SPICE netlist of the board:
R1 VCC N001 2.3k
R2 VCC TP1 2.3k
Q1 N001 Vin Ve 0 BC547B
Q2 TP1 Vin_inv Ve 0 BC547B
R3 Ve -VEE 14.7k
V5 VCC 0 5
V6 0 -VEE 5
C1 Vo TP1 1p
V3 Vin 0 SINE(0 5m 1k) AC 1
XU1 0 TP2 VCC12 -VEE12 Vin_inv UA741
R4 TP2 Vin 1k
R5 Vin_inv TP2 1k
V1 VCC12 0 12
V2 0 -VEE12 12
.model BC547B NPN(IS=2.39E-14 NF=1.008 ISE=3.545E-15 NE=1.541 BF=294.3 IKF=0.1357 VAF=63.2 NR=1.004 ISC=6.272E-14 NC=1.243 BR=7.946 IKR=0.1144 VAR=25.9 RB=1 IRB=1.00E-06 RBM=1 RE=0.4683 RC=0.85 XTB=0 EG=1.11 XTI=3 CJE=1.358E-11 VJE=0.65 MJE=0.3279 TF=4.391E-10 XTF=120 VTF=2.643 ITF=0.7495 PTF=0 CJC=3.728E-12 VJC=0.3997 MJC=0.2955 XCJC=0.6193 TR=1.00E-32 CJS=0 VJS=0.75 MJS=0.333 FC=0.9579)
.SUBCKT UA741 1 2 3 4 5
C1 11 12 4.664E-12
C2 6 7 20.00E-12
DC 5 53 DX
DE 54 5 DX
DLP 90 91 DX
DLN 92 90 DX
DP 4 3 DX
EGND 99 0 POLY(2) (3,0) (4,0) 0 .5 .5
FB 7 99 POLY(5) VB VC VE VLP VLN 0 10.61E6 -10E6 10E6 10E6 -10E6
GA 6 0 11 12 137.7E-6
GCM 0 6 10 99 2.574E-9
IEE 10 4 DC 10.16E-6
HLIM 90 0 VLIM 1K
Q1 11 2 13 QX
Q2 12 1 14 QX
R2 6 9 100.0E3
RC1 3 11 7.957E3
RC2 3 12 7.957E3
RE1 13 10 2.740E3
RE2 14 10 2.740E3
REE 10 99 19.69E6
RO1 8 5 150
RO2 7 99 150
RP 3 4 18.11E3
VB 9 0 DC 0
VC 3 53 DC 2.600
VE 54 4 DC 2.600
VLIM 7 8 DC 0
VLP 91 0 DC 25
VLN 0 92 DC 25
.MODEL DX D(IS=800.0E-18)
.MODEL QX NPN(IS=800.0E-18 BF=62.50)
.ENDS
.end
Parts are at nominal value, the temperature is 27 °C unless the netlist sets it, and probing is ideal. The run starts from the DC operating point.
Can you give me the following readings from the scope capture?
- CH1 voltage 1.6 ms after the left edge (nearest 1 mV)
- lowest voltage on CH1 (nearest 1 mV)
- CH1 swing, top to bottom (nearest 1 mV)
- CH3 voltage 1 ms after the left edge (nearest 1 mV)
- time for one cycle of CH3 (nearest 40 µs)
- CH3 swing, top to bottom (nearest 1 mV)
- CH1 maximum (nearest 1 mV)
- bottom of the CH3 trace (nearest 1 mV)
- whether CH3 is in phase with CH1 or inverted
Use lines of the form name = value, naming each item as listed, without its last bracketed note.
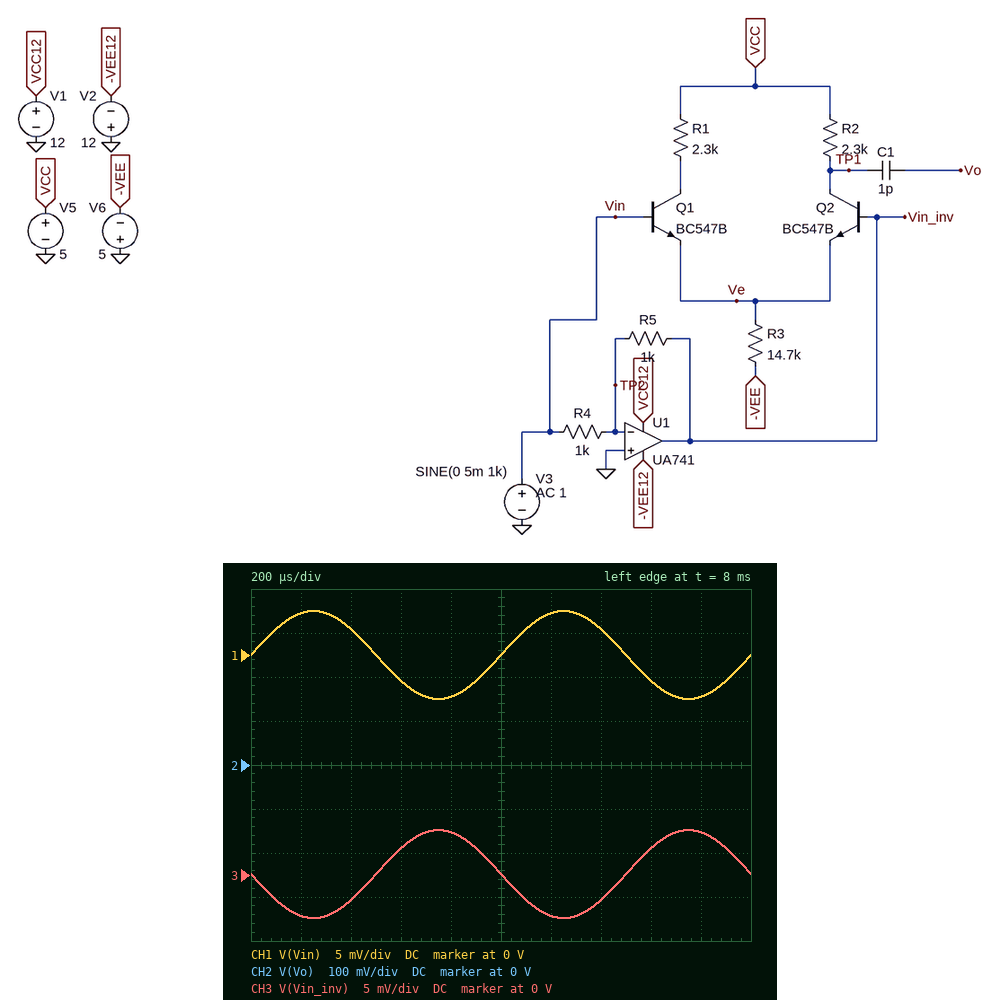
CH1 voltage 1.6 ms after the left edge = -3 mV
lowest voltage on CH1 = -5 mV
CH1 swing, top to bottom = 10 mV
CH3 voltage 1 ms after the left edge = 0 V
time for one cycle of CH3 = 1.00 ms
CH3 swing, top to bottom = 10 mV
CH1 maximum = 5 mV
bottom of the CH3 trace = -5 mV
whether CH3 is in phase with CH1 or inverted = inverted
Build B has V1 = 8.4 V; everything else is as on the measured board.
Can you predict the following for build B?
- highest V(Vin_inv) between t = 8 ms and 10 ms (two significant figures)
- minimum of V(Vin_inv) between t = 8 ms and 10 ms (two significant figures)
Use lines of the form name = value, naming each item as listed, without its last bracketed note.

highest V(Vin_inv) between t = 8 ms and 10 ms = 5.0 mV
minimum of V(Vin_inv) between t = 8 ms and 10 ms = -5.0 mV
